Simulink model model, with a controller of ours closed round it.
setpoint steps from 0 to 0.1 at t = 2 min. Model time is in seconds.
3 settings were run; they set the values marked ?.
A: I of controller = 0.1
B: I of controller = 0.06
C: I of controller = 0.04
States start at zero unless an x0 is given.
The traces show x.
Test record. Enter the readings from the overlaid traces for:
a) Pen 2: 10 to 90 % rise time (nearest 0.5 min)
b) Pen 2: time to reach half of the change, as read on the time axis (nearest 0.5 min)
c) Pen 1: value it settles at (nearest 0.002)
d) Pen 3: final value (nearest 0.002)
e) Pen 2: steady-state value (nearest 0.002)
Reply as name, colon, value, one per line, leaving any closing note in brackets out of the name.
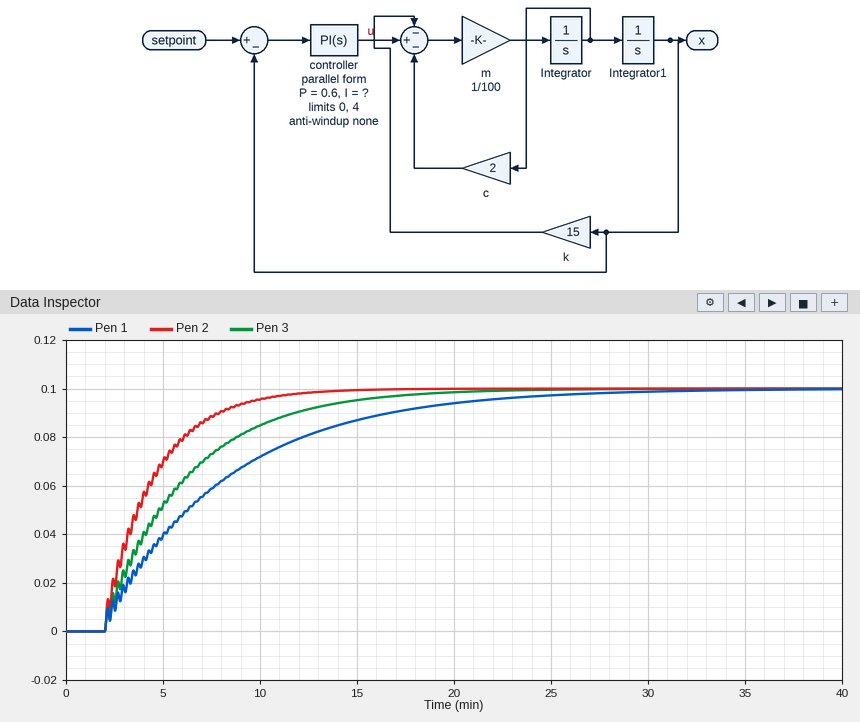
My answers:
Pen 2: 10 to 90 % rise time: 6.0 min
Pen 2: time to reach half of the change, as read on the time axis: 3.5 min
Pen 1: value it settles at: 0.100
Pen 3: final value: 0.100
Pen 2: steady-state value: 0.100
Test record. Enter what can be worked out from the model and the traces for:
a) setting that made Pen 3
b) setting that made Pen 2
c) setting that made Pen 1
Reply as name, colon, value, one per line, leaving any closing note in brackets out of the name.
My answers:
setting that made Pen 3: B
setting that made Pen 2: A
setting that made Pen 1: C
